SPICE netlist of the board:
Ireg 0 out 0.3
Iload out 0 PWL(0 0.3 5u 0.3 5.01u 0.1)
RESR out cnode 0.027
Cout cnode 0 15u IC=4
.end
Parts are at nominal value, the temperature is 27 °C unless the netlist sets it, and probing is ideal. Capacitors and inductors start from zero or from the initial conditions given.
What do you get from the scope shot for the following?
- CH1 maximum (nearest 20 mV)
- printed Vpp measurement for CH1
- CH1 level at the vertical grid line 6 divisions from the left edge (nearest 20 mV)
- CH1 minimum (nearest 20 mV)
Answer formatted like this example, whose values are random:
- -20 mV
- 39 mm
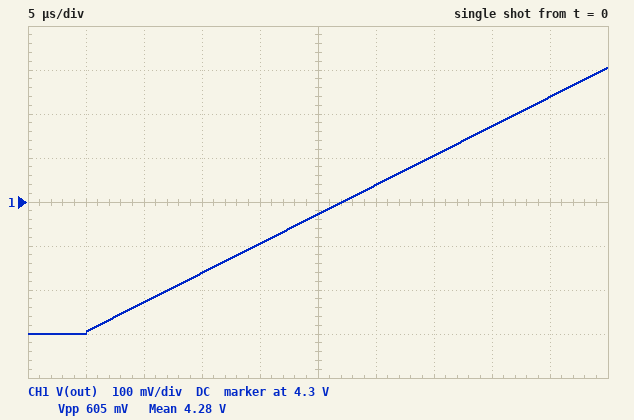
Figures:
- 4.60 V
- 605 mV
- 4.34 V
- 4.00 V
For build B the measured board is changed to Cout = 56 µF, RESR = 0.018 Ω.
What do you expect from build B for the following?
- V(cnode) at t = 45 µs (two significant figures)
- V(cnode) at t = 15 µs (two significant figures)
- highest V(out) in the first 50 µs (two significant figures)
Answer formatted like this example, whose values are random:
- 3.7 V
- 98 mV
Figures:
- 4.1 V
- 4.0 V
- 4.2 V
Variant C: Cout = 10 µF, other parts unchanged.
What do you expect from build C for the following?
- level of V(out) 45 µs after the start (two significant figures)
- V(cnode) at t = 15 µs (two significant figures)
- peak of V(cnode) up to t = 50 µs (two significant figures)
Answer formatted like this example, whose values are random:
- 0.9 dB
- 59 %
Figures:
- 4.8 V
- 4.2 V
- 4.9 V
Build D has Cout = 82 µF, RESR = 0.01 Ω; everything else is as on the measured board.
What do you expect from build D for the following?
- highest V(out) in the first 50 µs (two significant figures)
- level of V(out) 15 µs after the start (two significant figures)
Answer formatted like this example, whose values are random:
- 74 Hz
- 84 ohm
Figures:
- 4.1 V
- 4.0 V
